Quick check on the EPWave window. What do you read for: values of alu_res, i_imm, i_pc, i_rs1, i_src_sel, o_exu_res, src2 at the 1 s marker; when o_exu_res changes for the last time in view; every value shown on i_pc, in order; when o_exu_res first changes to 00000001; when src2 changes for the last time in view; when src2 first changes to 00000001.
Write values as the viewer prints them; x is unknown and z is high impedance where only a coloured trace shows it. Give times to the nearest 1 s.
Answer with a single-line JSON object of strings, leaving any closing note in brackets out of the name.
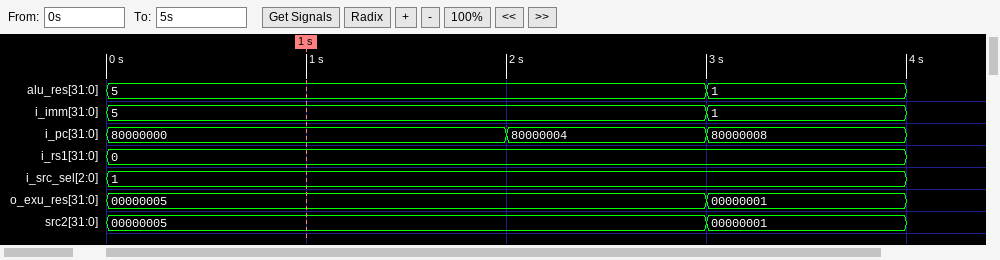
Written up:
{"values of alu_res, i_imm, i_pc, i_rs1, i_src_sel, o_exu_res, src2 at the 1 s marker": "alu_res=5, i_imm=5, i_pc=80000000, i_rs1=0, i_src_sel=1, o_exu_res=00000005, src2=00000005", "when o_exu_res changes for the last time in view": "3 s", "every value shown on i_pc, in order": "80000000, 80000004, 80000008", "when o_exu_res first changes to 00000001": "3 s", "when src2 changes for the last time in view": "3 s", "when src2 first changes to 00000001": "3 s"}
